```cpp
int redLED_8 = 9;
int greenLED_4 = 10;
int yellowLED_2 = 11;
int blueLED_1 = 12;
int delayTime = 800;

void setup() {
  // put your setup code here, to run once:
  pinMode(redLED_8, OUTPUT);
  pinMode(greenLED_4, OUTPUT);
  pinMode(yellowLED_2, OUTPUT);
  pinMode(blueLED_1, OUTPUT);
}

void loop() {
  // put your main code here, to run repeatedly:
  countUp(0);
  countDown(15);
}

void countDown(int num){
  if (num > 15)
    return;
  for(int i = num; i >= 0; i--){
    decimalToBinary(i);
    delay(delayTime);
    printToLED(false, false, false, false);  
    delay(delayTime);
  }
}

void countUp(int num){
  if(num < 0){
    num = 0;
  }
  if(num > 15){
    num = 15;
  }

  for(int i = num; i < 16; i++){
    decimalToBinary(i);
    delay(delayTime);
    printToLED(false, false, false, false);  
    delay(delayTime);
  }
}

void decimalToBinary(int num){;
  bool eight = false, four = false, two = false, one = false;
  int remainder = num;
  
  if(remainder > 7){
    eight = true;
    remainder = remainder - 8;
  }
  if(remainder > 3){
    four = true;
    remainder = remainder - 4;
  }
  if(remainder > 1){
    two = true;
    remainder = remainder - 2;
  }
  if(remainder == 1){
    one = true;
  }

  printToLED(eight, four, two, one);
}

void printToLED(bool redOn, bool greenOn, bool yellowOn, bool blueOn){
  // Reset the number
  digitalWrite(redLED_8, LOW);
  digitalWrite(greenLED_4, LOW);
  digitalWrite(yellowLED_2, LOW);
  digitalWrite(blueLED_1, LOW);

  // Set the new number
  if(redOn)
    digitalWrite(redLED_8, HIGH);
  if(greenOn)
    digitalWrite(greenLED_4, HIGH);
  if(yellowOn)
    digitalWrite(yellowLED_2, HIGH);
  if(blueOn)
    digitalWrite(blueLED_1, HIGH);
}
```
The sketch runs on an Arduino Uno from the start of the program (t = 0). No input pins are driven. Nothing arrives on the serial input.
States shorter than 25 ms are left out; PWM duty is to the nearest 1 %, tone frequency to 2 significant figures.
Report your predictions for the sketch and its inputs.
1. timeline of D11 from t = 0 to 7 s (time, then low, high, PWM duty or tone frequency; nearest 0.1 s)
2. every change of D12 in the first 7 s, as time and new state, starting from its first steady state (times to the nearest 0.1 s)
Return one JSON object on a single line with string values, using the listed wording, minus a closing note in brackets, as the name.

{"timeline of D11 from t = 0 to 7 s": "0 s low; 3.2 s high; 4 s low; 4.8 s high; 5.6 s low", "every change of D12 in the first 7 s, as time and new state, starting from its first steady state": "0 s low; 1.6 s high; 2.4 s low; 4.8 s high; 5.6 s low"}
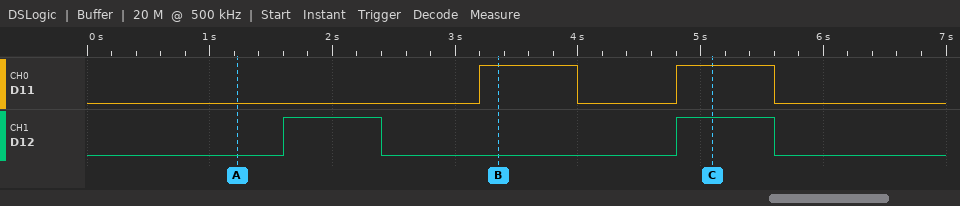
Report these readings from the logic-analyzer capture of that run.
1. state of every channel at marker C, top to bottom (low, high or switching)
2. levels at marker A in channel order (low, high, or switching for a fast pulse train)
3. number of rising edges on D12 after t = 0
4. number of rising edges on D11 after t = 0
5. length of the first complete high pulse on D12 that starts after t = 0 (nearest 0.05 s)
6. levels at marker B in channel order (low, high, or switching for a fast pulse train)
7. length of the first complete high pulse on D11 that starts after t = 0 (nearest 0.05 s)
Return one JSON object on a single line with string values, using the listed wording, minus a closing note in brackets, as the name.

{"state of every channel at marker C, top to bottom": "D11 high, D12 high", "levels at marker A in channel order": "D11 low, D12 low", "number of rising edges on D12 after t = 0": "2", "number of rising edges on D11 after t = 0": "2", "length of the first complete high pulse on D12 that starts after t = 0": "0.80 s", "levels at marker B in channel order": "D11 high, D12 low", "length of the first complete high pulse on D11 that starts after t = 0": "0.80 s"}
